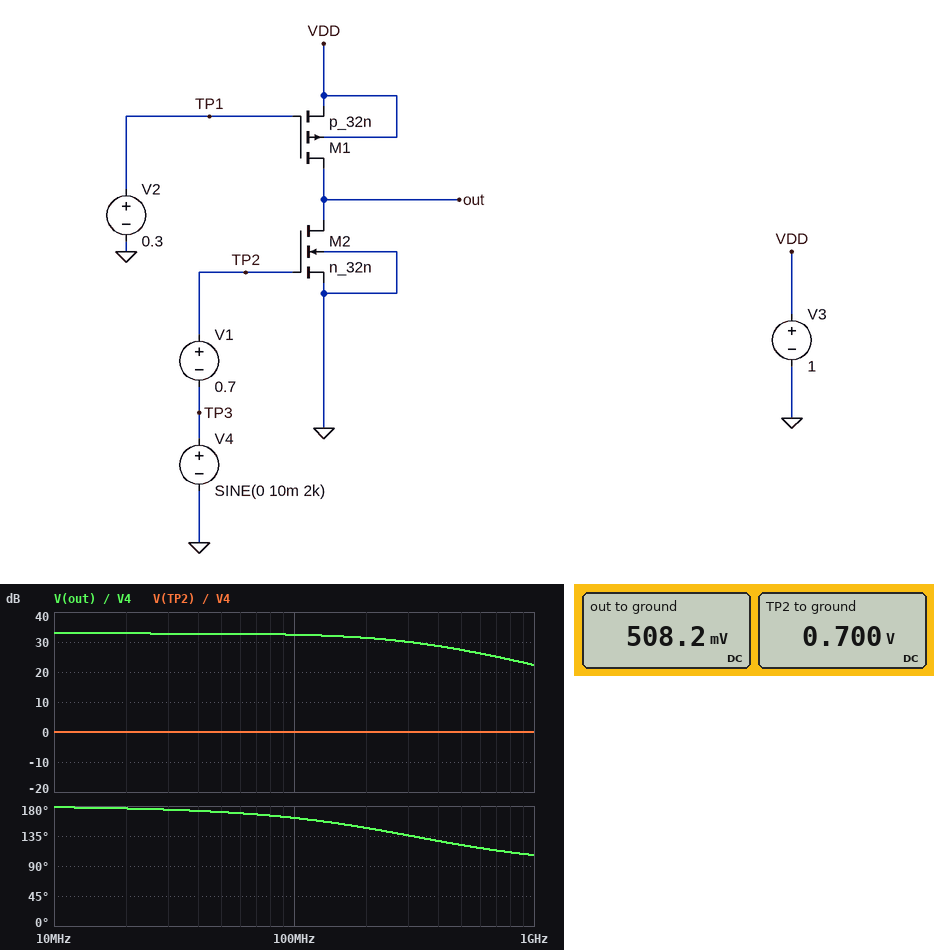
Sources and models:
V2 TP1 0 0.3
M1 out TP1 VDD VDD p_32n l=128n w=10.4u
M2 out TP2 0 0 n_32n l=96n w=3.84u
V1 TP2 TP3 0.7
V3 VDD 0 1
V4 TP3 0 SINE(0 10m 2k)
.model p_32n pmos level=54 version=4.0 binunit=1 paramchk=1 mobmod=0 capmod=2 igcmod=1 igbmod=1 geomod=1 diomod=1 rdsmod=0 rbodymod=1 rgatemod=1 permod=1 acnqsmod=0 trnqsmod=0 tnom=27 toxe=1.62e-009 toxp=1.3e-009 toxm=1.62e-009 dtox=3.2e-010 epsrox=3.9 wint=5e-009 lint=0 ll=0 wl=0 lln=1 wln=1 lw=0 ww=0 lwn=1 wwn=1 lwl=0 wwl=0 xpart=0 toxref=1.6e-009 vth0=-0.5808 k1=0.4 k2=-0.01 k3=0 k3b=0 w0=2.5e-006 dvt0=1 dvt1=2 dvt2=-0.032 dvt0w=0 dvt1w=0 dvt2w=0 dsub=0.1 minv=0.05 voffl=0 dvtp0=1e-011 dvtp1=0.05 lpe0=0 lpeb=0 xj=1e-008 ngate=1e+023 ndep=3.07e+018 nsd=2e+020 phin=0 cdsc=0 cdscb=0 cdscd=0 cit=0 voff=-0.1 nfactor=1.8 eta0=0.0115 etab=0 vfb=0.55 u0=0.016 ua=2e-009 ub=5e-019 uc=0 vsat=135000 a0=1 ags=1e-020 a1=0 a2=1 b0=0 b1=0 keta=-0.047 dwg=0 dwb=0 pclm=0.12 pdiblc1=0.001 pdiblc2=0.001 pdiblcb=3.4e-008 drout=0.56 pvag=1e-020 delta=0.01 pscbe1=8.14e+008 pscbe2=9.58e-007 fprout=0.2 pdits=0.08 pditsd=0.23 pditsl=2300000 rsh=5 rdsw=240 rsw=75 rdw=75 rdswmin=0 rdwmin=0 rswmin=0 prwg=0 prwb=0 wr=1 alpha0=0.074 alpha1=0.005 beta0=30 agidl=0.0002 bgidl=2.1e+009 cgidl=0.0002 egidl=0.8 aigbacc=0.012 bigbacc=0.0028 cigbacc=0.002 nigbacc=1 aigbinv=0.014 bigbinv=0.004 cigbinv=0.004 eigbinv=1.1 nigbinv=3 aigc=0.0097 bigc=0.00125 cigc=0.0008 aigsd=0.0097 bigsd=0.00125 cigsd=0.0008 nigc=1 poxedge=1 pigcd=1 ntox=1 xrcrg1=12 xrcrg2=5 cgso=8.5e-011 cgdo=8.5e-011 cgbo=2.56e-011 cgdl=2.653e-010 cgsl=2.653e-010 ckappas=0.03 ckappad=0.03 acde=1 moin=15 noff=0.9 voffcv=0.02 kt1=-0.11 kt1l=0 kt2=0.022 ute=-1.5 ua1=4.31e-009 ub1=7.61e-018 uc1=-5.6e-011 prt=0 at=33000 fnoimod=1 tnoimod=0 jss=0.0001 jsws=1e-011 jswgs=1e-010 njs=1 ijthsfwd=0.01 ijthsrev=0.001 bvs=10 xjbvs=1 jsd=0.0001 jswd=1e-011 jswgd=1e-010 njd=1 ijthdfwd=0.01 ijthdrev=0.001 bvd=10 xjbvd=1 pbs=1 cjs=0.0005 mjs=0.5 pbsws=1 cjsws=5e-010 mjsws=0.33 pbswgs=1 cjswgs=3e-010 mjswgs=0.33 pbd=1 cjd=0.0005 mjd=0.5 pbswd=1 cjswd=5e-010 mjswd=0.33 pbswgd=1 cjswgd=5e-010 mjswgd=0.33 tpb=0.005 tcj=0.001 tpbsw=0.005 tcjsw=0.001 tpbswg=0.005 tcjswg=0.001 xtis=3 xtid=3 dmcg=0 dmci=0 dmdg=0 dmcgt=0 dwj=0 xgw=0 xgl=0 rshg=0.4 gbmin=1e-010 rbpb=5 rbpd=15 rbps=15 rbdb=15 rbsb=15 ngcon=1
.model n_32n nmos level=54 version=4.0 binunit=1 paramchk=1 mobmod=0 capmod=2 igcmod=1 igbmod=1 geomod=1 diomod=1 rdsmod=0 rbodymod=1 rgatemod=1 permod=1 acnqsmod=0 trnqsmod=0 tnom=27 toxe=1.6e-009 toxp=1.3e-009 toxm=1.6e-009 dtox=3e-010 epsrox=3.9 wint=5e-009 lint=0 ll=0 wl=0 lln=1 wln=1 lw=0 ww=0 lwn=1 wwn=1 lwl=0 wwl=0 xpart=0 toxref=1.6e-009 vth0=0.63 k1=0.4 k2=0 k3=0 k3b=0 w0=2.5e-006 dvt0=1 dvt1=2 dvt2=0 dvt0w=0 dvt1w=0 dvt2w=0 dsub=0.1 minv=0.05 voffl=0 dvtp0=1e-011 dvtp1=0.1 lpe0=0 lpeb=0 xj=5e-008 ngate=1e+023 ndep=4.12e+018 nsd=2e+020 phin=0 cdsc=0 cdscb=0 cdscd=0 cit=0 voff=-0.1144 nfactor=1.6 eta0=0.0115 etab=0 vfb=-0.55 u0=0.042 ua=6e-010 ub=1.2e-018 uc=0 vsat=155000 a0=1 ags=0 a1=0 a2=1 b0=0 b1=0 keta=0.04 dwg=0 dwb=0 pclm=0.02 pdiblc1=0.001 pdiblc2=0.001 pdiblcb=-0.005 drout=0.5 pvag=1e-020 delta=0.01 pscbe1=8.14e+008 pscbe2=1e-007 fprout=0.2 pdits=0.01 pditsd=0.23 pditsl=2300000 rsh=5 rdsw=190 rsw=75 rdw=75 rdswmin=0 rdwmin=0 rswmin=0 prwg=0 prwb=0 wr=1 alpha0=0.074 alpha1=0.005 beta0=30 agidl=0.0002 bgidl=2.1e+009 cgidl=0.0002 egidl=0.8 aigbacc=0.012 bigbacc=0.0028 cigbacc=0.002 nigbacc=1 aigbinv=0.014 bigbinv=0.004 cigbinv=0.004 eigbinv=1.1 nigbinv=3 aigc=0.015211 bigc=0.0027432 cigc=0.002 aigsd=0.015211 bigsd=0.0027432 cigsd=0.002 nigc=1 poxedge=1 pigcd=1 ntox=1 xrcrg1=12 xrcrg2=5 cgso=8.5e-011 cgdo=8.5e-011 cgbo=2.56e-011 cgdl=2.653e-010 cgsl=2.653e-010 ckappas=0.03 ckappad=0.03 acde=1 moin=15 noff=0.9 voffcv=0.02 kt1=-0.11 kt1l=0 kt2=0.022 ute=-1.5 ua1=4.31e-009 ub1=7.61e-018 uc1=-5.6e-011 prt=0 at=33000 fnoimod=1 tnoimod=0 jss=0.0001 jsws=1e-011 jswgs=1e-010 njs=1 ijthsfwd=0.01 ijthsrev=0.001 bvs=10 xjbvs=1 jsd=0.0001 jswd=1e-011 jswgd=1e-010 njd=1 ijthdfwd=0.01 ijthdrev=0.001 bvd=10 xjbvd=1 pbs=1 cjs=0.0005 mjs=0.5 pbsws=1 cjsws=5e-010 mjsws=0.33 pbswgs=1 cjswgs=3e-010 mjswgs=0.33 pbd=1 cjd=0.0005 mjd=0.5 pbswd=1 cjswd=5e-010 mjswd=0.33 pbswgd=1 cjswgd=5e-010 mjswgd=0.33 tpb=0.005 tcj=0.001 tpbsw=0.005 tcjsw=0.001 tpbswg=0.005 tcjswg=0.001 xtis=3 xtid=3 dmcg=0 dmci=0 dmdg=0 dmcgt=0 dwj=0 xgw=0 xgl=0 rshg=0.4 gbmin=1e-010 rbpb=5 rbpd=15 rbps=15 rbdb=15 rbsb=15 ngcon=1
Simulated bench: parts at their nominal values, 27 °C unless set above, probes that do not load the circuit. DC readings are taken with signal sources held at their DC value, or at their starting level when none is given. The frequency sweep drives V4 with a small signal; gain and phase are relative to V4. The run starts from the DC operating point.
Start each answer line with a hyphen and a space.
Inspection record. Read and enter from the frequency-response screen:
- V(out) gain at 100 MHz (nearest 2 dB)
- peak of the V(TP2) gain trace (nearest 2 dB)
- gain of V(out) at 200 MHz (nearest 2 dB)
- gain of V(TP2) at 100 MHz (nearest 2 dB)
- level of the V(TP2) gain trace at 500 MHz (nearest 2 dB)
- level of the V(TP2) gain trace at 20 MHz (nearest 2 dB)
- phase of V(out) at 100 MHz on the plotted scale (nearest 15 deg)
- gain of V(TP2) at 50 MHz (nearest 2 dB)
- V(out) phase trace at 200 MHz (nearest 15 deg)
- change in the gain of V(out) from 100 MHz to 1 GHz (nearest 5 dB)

- 32 dB
- 0 dB
- 32 dB
- 0 dB
- 0 dB
- 0 dB
- 165 deg
- 0 dB
- 150 deg
- -10 dB
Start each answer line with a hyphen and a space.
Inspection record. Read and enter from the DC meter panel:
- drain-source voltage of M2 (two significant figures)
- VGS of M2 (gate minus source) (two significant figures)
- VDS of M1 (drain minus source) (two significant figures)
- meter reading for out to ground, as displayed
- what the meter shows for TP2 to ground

- 510 mV
- 700 mV
- -490 mV
- 508.2 mV
- 0.700 V
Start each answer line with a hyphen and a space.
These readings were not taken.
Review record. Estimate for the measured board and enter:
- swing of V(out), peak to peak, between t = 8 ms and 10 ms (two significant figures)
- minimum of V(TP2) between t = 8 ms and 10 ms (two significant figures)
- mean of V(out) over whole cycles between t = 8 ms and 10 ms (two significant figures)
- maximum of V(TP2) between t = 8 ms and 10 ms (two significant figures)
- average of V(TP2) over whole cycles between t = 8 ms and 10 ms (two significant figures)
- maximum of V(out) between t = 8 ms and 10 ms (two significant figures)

- 680 mV
- 690 mV
- 500 mV
- 710 mV
- 700 mV
- 840 mV
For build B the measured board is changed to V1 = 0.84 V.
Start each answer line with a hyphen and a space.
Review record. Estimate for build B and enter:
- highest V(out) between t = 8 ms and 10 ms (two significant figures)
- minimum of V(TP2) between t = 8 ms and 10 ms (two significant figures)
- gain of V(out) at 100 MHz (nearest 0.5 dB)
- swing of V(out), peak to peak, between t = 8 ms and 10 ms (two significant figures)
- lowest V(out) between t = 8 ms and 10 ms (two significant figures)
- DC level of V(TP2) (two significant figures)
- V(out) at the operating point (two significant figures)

- 35 mV
- 830 mV
- -16.5 dB
- 3.0 mV
- 32 mV
- 840 mV
- 33 mV
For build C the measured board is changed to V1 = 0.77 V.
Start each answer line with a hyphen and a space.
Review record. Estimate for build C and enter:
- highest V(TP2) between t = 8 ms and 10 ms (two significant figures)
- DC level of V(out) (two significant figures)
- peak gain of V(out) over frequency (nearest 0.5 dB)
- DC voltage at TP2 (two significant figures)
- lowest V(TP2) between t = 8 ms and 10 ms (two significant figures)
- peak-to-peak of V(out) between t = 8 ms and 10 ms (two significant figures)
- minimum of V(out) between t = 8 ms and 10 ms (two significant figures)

- 780 mV
- 51 mV
- -7.5 dB
- 770 mV
- 760 mV
- 8.5 mV
- 47 mV
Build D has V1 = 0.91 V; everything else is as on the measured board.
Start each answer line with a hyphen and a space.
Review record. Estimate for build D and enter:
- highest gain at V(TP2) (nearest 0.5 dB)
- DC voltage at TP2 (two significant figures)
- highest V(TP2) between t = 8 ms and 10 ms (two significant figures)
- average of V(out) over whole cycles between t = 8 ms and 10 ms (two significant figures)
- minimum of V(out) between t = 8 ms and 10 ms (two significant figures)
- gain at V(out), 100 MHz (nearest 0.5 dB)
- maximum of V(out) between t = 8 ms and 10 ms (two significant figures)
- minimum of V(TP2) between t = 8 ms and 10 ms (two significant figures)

- 0 dB
- 910 mV
- 920 mV
- 26 mV
- 25 mV
- -22.5 dB
- 27 mV
- 900 mV
